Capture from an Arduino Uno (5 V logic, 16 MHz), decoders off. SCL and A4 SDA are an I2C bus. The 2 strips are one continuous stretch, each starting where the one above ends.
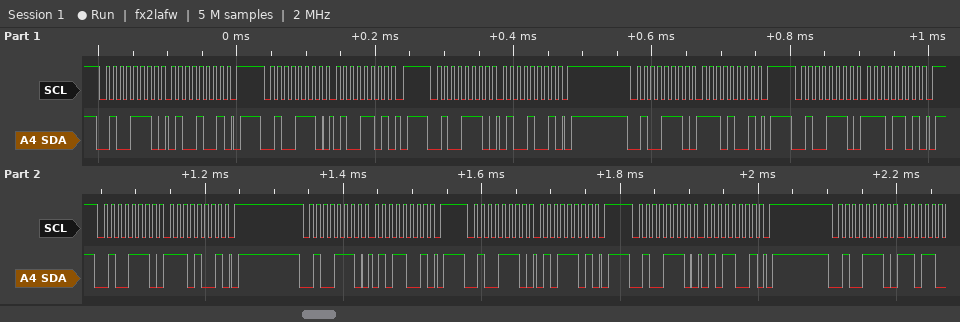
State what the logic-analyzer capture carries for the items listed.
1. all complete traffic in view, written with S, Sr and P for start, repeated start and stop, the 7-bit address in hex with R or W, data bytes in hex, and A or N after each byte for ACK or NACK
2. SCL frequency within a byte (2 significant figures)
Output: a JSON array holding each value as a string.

["S 27W A 49 A P S 27W A 4D A P S 27W A 49 A P S 27W A E9 A P S 27W A ED A P S 27W A E9 A P S 27W A 59 A P S 27W A 5D A P S 27W A 59 A P S 27W A", "100 kHz"]
